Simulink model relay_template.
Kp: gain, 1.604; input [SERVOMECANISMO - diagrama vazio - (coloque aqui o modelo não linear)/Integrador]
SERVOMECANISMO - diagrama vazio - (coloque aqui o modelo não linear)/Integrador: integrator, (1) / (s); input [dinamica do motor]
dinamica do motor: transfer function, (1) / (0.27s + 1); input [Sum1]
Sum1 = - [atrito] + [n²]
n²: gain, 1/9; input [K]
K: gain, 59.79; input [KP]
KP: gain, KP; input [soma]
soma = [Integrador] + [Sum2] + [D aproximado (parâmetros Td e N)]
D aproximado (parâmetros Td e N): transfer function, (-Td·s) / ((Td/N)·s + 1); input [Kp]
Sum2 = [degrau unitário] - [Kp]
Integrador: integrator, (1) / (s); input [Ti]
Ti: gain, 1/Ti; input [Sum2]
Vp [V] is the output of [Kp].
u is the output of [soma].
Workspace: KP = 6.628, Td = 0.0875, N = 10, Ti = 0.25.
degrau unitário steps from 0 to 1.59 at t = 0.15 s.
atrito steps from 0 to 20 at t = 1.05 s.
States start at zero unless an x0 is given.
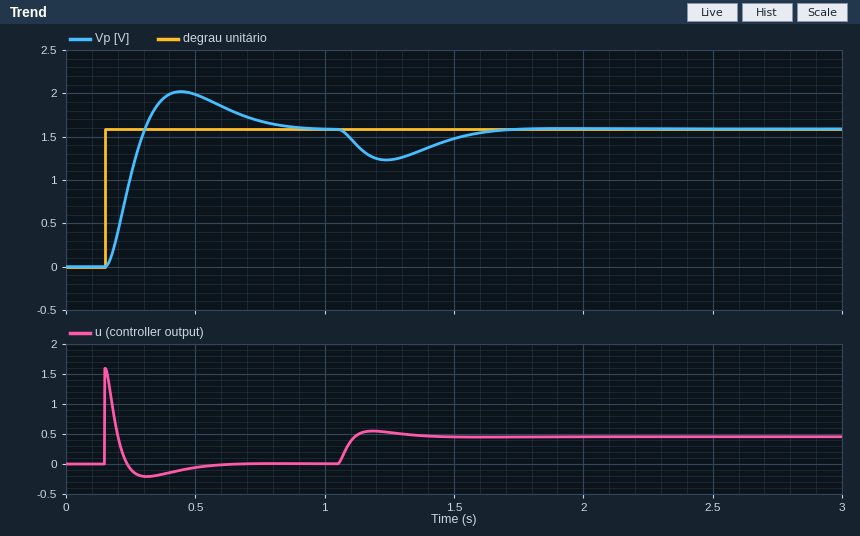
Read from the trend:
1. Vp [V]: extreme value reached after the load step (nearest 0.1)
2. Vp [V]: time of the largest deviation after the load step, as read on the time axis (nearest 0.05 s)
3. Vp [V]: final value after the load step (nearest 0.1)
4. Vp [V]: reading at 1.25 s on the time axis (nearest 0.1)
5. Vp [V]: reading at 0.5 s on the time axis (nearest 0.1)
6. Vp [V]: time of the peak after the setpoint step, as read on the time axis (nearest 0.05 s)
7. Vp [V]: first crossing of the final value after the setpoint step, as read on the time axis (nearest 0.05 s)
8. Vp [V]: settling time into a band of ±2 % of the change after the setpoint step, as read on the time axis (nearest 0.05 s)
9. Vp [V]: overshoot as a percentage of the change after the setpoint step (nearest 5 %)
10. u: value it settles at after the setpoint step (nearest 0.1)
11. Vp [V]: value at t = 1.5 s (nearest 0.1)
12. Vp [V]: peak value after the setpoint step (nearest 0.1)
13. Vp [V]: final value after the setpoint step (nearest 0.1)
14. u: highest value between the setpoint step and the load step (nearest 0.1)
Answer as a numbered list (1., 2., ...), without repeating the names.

1. 1.2
2. 1.25 s
3. 1.6
4. 1.2
5. 2.0
6. 0.45 s
7. 0.30 s
8. 0.85 s
9. 25 %
10. 0.0
11. 1.5
12. 2.0
13. 1.6
14. 1.6
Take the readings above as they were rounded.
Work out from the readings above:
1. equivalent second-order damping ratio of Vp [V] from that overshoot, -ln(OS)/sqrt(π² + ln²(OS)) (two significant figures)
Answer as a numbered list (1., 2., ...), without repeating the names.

1. 0.40
